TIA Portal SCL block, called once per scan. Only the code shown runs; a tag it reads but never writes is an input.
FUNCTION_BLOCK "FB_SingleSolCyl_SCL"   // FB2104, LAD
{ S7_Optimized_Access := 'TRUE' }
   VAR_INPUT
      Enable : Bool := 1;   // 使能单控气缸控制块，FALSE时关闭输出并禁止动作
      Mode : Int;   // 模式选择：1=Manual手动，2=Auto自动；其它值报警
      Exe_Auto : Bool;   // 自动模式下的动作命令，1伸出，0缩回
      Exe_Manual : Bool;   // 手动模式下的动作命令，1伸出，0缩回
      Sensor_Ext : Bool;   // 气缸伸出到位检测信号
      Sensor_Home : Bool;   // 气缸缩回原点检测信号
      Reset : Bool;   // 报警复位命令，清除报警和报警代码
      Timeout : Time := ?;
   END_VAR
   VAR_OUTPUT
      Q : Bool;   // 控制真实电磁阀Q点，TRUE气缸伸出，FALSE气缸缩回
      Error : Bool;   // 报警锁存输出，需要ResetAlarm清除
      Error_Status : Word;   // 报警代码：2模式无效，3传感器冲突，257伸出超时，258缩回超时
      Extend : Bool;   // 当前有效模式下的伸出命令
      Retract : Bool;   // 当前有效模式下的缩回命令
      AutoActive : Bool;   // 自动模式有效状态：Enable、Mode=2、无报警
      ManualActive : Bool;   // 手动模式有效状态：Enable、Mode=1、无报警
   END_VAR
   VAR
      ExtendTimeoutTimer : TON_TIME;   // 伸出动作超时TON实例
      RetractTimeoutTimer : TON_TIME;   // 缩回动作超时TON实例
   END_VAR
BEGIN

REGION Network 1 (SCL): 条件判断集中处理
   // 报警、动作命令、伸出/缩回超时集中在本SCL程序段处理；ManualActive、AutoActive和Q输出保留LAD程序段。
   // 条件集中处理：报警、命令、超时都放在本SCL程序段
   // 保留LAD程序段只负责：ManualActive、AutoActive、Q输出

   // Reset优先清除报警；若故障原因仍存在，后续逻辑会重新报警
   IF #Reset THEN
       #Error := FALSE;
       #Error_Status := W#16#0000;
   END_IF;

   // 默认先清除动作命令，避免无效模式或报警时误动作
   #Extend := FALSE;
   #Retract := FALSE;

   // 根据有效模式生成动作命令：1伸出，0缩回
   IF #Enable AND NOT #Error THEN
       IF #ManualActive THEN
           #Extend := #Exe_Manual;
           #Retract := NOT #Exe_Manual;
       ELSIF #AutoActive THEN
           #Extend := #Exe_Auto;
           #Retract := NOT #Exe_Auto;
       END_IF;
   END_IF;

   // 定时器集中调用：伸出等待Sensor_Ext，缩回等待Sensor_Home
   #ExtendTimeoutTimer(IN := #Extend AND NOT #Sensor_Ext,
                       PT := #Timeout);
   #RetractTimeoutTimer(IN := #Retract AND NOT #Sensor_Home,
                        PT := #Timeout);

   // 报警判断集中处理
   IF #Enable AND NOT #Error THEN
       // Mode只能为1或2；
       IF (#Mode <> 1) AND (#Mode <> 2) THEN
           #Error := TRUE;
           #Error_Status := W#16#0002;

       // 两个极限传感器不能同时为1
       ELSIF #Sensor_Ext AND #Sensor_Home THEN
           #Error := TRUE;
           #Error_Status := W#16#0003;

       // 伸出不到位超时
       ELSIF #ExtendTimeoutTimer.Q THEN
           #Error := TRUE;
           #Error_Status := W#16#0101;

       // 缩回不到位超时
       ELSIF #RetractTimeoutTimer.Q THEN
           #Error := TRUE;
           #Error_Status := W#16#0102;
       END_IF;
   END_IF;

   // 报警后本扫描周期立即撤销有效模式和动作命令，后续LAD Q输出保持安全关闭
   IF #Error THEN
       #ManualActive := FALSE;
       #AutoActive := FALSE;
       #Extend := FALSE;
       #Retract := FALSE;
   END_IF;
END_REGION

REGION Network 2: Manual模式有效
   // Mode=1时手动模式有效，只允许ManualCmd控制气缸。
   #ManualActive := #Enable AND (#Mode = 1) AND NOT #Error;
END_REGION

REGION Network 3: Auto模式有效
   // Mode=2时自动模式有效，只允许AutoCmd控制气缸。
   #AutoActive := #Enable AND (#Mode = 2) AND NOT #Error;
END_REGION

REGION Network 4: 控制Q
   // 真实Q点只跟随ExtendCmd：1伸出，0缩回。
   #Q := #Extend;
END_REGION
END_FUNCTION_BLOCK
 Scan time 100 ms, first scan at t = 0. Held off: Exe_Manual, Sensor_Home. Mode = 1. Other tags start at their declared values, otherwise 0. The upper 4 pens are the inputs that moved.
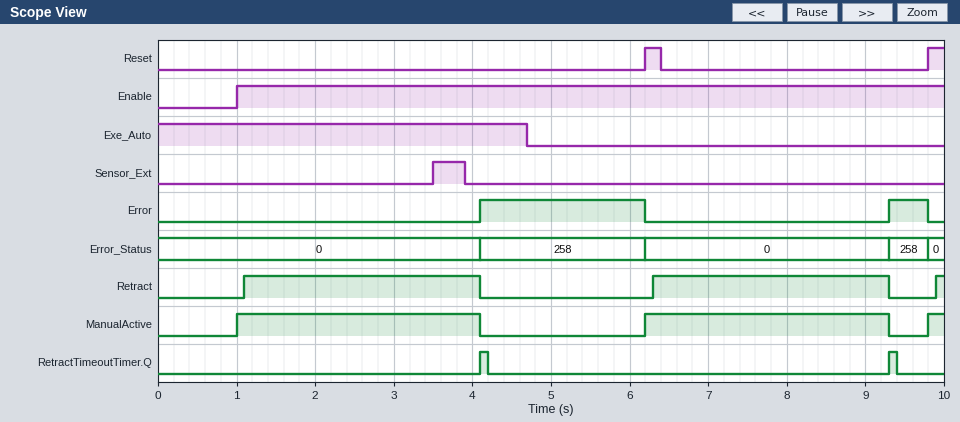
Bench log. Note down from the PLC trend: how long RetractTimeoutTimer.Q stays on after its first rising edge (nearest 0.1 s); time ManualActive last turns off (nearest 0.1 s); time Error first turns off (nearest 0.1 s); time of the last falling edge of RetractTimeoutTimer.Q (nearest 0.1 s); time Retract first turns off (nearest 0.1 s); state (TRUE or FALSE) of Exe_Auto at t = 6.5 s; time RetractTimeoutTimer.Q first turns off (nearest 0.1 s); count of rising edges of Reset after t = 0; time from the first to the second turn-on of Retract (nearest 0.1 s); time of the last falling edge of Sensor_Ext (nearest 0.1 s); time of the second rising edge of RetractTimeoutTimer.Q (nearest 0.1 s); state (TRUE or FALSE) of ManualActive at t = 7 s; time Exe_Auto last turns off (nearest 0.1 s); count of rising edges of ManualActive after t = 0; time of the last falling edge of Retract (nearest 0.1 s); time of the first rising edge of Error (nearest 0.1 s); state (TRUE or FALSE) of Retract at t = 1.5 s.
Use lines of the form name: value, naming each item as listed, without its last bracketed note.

how long RetractTimeoutTimer.Q stays on after its first rising edge: 0.1 s
time ManualActive last turns off: 9.3 s
time Error first turns off: 6.2 s
time of the last falling edge of RetractTimeoutTimer.Q: 9.4 s
time Retract first turns off: 4.1 s
state (TRUE or FALSE) of Exe_Auto at t = 6.5 s: FALSE
time RetractTimeoutTimer.Q first turns off: 4.2 s
count of rising edges of Reset after t = 0: 2
time from the first to the second turn-on of Retract: 5.2 s
time of the last falling edge of Sensor_Ext: 3.9 s
time of the second rising edge of RetractTimeoutTimer.Q: 9.3 s
state (TRUE or FALSE) of ManualActive at t = 7 s: TRUE
time Exe_Auto last turns off: 4.7 s
count of rising edges of ManualActive after t = 0: 3
time of the last falling edge of Retract: 9.3 s
time of the first rising edge of Error: 4.1 s
state (TRUE or FALSE) of Retract at t = 1.5 s: TRUE
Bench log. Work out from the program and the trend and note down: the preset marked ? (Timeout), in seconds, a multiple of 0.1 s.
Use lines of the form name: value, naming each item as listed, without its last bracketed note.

the preset marked ? (Timeout), in seconds, a multiple of 0.1 s: 3.0 s
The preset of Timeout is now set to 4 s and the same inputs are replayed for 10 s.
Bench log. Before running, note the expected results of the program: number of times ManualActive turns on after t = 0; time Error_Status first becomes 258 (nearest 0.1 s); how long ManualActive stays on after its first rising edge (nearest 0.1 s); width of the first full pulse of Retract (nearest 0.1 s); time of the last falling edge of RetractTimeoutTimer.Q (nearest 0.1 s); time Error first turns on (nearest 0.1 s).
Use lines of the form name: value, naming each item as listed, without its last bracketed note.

number of times ManualActive turns on after t = 0: 2
time Error_Status first becomes 258: 5.1 s
how long ManualActive stays on after its first rising edge: 4.1 s
width of the first full pulse of Retract: 4.0 s
time of the last falling edge of RetractTimeoutTimer.Q: 5.2 s
time Error first turns on: 5.1 s
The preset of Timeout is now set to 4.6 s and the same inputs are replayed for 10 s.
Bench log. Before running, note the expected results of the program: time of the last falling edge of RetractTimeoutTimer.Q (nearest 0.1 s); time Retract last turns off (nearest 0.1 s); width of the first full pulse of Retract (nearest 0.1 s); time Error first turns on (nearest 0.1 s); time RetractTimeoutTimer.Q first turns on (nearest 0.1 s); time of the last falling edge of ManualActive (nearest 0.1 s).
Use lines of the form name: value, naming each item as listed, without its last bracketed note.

time of the last falling edge of RetractTimeoutTimer.Q: 5.8 s
time Retract last turns off: 5.7 s
width of the first full pulse of Retract: 4.6 s
time Error first turns on: 5.7 s
time RetractTimeoutTimer.Q first turns on: 5.7 s
time of the last falling edge of ManualActive: 5.7 s
